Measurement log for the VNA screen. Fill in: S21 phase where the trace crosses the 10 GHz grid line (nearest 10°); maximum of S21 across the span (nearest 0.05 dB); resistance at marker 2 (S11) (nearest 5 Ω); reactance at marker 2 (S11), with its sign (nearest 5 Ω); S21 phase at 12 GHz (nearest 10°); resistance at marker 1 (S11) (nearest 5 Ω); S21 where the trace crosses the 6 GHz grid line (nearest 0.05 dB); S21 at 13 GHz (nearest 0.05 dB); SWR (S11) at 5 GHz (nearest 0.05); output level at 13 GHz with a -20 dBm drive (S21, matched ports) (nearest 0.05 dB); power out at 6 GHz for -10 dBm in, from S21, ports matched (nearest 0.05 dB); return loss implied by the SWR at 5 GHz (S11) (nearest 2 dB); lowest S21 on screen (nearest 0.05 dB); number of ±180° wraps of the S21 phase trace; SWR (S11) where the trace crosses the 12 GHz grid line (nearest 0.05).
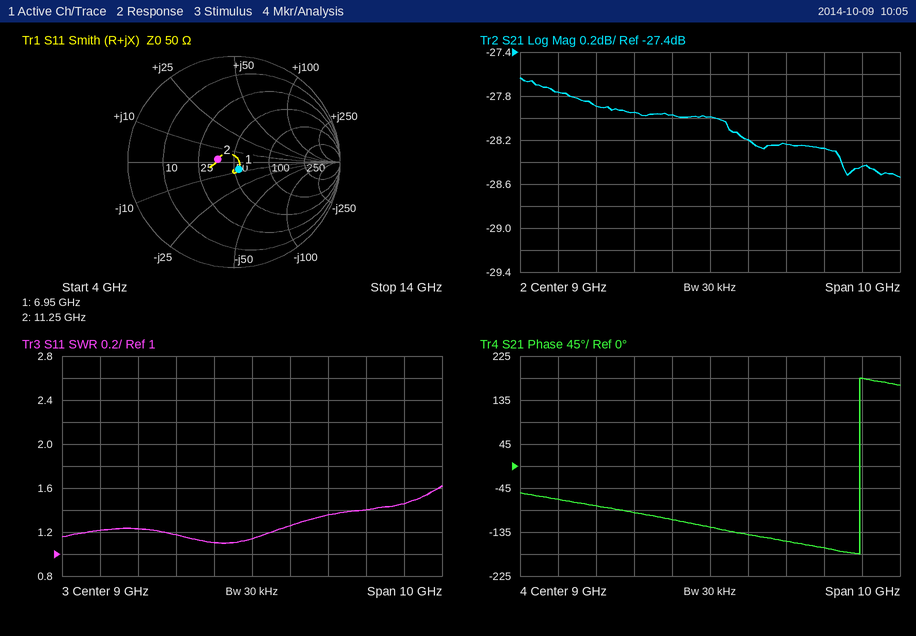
-140°
-27.65 dB
35 Ω
0 Ω
-170°
55 Ω
-27.90 dB
-28.45 dB
1.20
-48.45 dBm
-37.90 dBm
20 dB
-28.55 dB
1
1.40
